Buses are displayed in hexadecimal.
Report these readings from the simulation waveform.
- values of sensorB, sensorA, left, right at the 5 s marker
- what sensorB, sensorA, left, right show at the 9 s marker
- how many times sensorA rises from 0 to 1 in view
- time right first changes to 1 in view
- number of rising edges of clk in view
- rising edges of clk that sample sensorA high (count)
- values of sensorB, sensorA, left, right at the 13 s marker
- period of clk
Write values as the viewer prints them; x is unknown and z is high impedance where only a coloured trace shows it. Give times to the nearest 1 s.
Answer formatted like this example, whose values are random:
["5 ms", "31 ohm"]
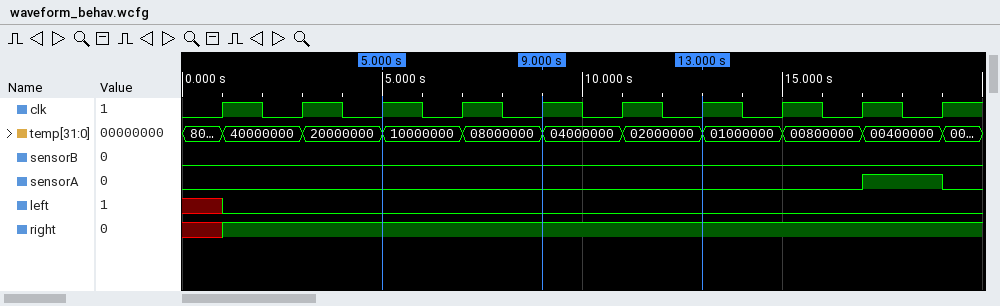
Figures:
["sensorB=0, sensorA=0, left=0, right=1", "sensorB=0, sensorA=0, left=0, right=1", "1", "1 s", "10", "1", "sensorB=0, sensorA=0, left=0, right=1", "2 s"]
